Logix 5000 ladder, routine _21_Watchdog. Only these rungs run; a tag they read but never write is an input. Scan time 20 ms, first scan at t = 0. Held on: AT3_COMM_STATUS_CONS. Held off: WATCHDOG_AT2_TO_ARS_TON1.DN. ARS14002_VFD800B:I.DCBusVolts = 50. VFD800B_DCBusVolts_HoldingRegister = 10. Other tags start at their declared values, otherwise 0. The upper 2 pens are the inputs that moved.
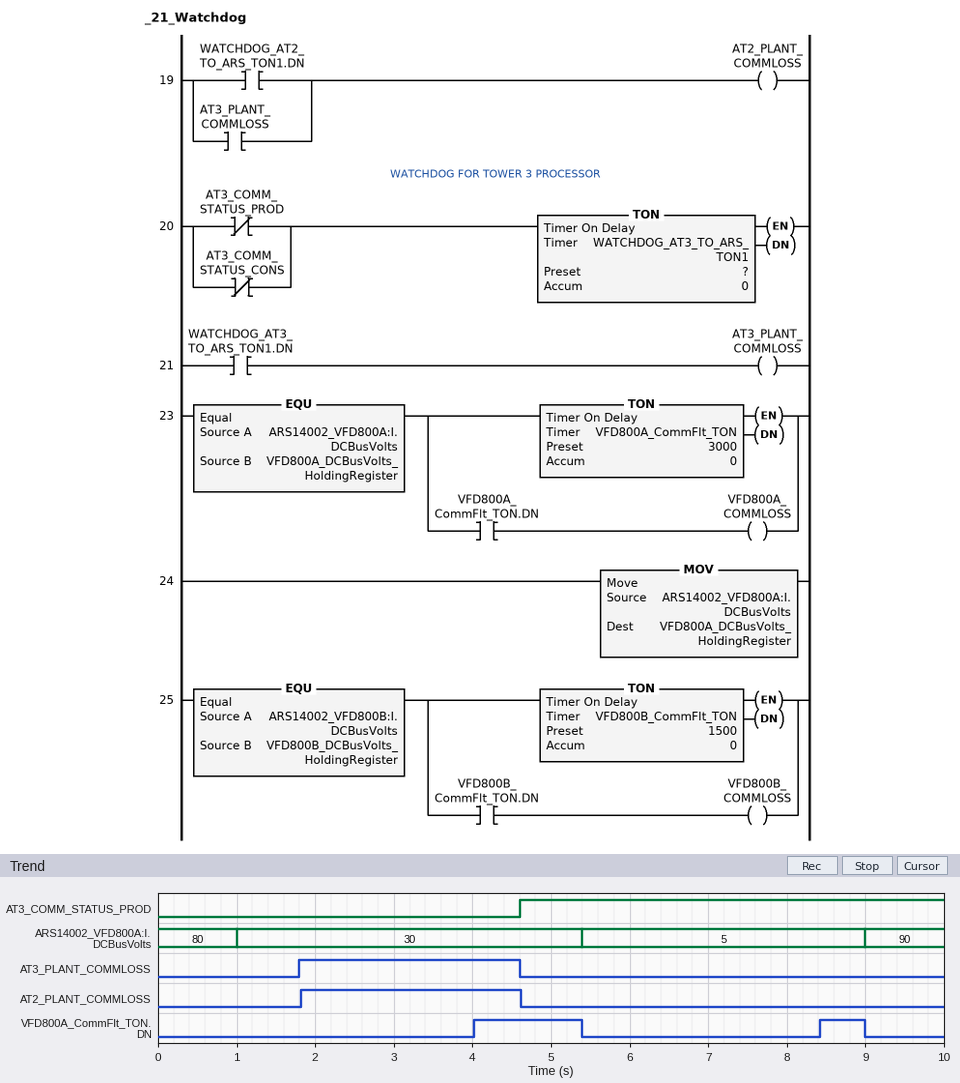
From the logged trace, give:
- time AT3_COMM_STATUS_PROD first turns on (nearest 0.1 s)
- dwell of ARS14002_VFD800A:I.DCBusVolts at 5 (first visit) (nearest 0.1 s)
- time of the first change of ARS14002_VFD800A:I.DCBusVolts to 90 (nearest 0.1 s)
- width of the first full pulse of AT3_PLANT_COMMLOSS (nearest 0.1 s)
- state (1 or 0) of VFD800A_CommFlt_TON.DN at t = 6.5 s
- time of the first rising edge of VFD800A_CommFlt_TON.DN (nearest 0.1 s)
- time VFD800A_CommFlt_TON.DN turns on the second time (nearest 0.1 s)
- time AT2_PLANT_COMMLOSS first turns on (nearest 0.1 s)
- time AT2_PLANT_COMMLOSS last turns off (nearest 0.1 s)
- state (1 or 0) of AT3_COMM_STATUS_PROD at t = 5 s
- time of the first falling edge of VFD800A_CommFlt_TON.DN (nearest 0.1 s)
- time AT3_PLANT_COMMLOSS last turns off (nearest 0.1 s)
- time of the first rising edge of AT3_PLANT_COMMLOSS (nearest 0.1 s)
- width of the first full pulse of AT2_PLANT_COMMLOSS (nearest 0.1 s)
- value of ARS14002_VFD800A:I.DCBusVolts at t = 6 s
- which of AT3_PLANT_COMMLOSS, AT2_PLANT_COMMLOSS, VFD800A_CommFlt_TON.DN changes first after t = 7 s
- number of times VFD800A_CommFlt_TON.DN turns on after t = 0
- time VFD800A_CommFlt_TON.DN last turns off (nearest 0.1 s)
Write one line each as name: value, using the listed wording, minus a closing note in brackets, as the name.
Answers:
time AT3_COMM_STATUS_PROD first turns on: 4.6 s
dwell of ARS14002_VFD800A:I.DCBusVolts at 5 (first visit): 3.6 s
time of the first change of ARS14002_VFD800A:I.DCBusVolts to 90: 9.0 s
width of the first full pulse of AT3_PLANT_COMMLOSS: 2.8 s
state (1 or 0) of VFD800A_CommFlt_TON.DN at t = 6.5 s: 0
time of the first rising edge of VFD800A_CommFlt_TON.DN: 4.0 s
time VFD800A_CommFlt_TON.DN turns on the second time: 8.4 s
time AT2_PLANT_COMMLOSS first turns on: 1.8 s
time AT2_PLANT_COMMLOSS last turns off: 4.6 s
state (1 or 0) of AT3_COMM_STATUS_PROD at t = 5 s: 1
time of the first falling edge of VFD800A_CommFlt_TON.DN: 5.4 s
time AT3_PLANT_COMMLOSS last turns off: 4.6 s
time of the first rising edge of AT3_PLANT_COMMLOSS: 1.8 s
width of the first full pulse of AT2_PLANT_COMMLOSS: 2.8 s
value of ARS14002_VFD800A:I.DCBusVolts at t = 6 s: 5
which of AT3_PLANT_COMMLOSS, AT2_PLANT_COMMLOSS, VFD800A_CommFlt_TON.DN changes first after t = 7 s: VFD800A_CommFlt_TON.DN
number of times VFD800A_CommFlt_TON.DN turns on after t = 0: 2
time VFD800A_CommFlt_TON.DN last turns off: 9.0 s
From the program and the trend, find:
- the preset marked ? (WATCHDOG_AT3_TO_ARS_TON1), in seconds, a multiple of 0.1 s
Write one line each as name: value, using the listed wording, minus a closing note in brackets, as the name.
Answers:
the preset marked ? (WATCHDOG_AT3_TO_ARS_TON1), in seconds, a multiple of 0.1 s: 1.8 s
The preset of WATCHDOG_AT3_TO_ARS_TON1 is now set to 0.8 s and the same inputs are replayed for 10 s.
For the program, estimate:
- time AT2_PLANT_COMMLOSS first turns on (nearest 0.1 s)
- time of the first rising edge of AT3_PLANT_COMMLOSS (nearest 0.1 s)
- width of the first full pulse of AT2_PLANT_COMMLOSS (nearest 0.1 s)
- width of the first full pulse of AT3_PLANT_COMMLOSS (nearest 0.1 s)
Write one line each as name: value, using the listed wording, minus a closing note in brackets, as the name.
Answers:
time AT2_PLANT_COMMLOSS first turns on: 0.8 s
time of the first rising edge of AT3_PLANT_COMMLOSS: 0.8 s
width of the first full pulse of AT2_PLANT_COMMLOSS: 3.8 s
width of the first full pulse of AT3_PLANT_COMMLOSS: 3.8 s
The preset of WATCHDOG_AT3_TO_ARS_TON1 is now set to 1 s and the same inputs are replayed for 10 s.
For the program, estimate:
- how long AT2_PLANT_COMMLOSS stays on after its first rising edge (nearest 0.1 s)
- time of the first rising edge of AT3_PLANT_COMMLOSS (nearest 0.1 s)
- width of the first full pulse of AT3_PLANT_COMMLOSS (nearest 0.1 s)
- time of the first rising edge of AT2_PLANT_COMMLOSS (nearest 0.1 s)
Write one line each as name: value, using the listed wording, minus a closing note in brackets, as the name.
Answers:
how long AT2_PLANT_COMMLOSS stays on after its first rising edge: 3.6 s
time of the first rising edge of AT3_PLANT_COMMLOSS: 1.0 s
width of the first full pulse of AT3_PLANT_COMMLOSS: 3.6 s
time of the first rising edge of AT2_PLANT_COMMLOSS: 1.0 s
